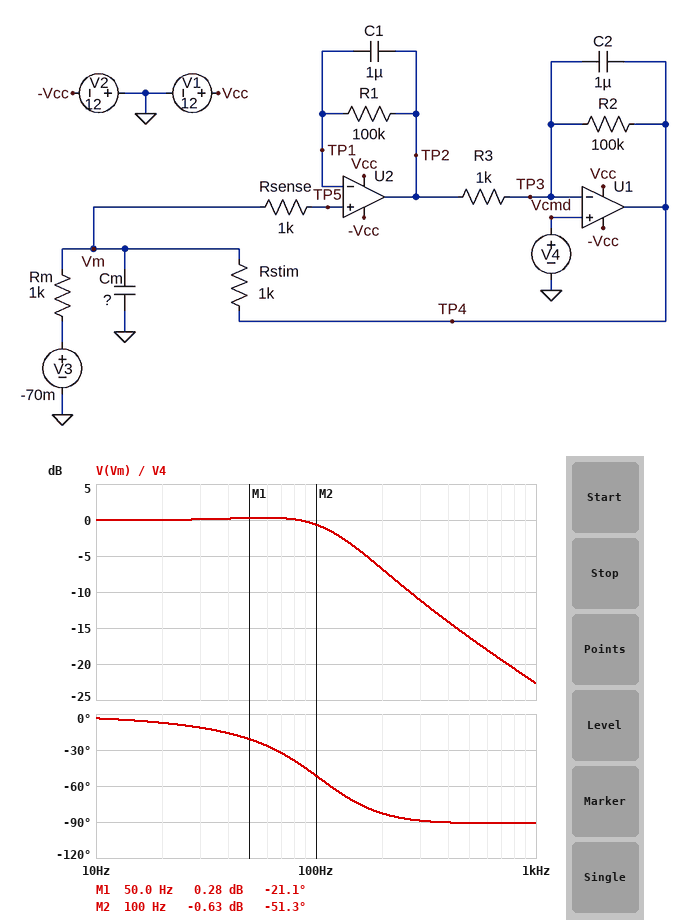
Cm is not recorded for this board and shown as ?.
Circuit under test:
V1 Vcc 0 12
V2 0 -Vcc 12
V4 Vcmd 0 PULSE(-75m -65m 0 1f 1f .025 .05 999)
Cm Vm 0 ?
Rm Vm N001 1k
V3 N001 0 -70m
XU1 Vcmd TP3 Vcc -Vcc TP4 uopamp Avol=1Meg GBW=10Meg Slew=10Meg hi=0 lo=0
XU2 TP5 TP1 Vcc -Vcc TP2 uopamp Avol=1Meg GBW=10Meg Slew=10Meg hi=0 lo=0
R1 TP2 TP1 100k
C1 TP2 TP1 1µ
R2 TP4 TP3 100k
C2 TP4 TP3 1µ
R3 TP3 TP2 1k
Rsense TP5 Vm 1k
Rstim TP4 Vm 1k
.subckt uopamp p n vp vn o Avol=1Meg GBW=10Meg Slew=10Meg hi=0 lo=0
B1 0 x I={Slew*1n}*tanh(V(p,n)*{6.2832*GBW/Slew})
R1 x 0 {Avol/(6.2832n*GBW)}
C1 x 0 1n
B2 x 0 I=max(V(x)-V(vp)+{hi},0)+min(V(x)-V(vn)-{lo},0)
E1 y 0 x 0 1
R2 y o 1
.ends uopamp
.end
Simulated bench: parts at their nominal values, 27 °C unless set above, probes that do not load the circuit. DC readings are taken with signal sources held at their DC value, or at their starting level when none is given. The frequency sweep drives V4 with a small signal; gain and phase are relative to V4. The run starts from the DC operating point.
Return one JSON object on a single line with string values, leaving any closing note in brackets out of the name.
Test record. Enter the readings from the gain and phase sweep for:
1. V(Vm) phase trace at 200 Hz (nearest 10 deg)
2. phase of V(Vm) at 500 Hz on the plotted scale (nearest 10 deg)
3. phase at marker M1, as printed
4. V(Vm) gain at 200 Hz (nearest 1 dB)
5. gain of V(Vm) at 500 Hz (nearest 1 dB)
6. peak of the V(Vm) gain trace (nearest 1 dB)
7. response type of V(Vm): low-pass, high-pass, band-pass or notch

{"V(Vm) phase trace at 200 Hz": "-80 deg", "phase of V(Vm) at 500 Hz on the plotted scale": "-90 deg", "phase at marker M1, as printed": "-21.1 deg", "V(Vm) gain at 200 Hz": "-7 dB", "gain of V(Vm) at 500 Hz": "-16 dB", "peak of the V(Vm) gain trace": "0 dB", "response type of V(Vm): low-pass, high-pass, band-pass or notch": "low-pass"}
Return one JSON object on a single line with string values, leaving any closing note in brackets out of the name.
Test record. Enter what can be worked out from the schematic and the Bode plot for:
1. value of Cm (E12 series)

{"value of Cm": "2.2 µF"}
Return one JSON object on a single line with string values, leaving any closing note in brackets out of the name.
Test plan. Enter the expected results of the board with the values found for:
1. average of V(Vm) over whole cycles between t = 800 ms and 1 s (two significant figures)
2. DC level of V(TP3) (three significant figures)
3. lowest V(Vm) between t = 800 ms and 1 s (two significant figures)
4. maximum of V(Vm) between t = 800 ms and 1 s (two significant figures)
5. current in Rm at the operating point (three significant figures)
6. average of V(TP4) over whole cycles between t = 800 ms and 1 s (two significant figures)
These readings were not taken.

{"average of V(Vm) over whole cycles between t = 800 ms and 1 s": "-70 mV", "DC level of V(TP3)": "-75.0 mV", "lowest V(Vm) between t = 800 ms and 1 s": "-76 mV", "maximum of V(Vm) between t = 800 ms and 1 s": "-64 mV", "current in Rm at the operating point": "4.95 µA", "average of V(TP4) over whole cycles between t = 800 ms and 1 s": "-70 mV"}
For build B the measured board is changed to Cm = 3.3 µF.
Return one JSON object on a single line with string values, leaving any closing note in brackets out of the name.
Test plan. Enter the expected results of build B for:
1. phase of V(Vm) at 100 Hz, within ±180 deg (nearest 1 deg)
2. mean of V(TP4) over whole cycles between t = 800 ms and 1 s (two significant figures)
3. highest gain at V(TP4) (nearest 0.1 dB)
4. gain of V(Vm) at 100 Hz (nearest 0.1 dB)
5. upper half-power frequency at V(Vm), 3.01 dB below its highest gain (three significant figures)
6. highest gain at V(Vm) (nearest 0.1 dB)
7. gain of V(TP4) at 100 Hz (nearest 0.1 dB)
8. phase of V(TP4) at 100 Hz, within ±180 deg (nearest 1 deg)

{"phase of V(Vm) at 100 Hz, within ±180 deg": "-71 deg", "mean of V(TP4) over whole cycles between t = 800 ms and 1 s": "-70 mV", "highest gain at V(TP4)": "9.0 dB", "gain of V(Vm) at 100 Hz": "-0.8 dB", "upper half-power frequency at V(Vm), 3.01 dB below its highest gain": "110 Hz", "highest gain at V(Vm)": "1.2 dB", "gain of V(TP4) at 100 Hz": "8.4 dB", "phase of V(TP4) at 100 Hz, within ±180 deg": "-25 deg"}
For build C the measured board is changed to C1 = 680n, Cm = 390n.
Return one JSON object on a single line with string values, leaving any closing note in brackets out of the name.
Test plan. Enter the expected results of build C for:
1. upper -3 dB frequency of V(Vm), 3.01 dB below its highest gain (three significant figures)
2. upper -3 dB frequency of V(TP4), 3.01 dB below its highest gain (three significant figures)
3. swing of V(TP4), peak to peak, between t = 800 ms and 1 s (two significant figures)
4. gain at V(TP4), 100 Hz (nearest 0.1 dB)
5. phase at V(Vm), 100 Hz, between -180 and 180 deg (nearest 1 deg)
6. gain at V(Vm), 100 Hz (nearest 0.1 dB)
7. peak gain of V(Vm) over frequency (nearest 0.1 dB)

{"upper -3 dB frequency of V(Vm), 3.01 dB below its highest gain": "142 Hz", "upper -3 dB frequency of V(TP4), 3.01 dB below its highest gain": "150 Hz", "swing of V(TP4), peak to peak, between t = 800 ms and 1 s": "20 mV", "gain at V(TP4), 100 Hz": "3.9 dB", "phase at V(Vm), 100 Hz, between -180 and 180 deg": "-24 deg", "gain at V(Vm), 100 Hz": "-2.2 dB", "peak gain of V(Vm) over frequency": "-0.1 dB"}
